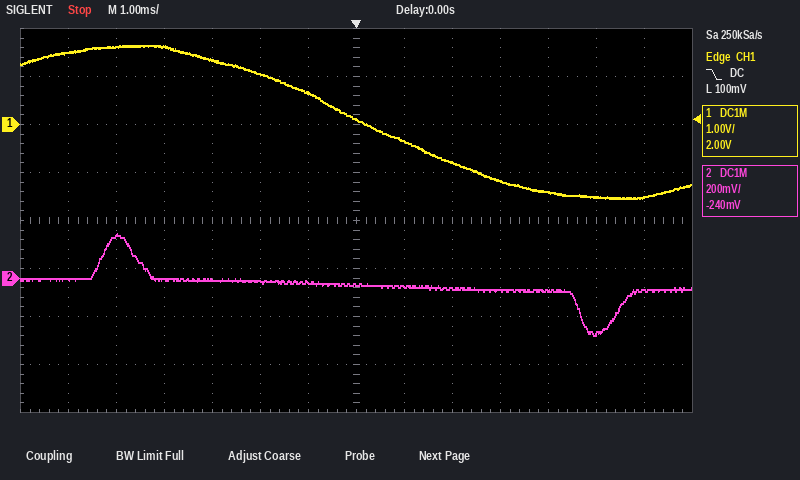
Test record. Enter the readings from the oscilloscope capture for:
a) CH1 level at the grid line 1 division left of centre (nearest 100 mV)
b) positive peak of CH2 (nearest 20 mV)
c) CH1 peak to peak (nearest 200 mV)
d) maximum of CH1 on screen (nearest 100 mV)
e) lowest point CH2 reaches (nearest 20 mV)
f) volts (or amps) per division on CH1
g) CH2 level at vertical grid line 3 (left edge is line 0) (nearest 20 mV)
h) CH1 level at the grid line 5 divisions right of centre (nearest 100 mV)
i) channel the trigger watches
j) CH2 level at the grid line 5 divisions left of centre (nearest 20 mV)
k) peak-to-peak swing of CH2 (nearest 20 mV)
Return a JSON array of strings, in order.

["700 mV", "180 mV", "3.2 V", "1.6 V", "-240 mV", "1 V", "0 mV", "-1.5 V", "CH1", "180 mV", "420 mV"]
